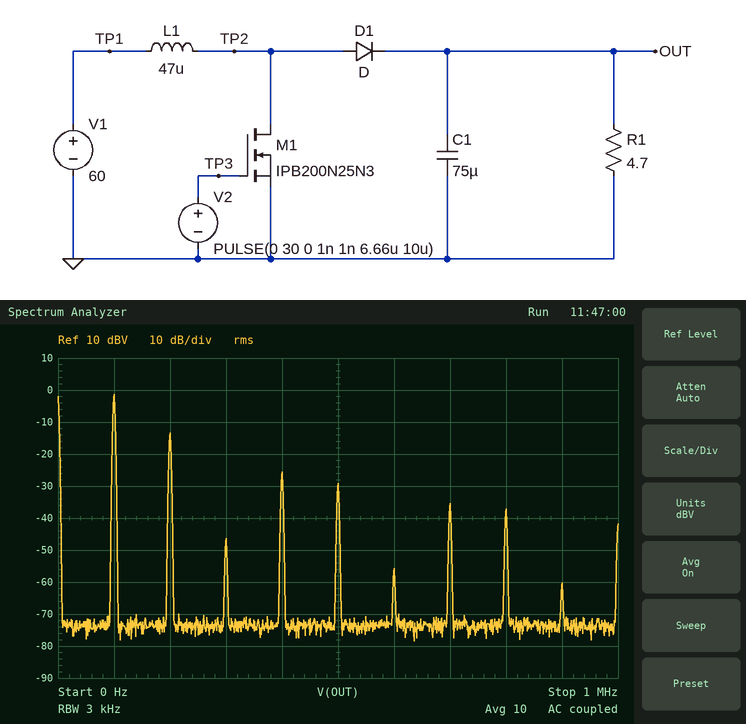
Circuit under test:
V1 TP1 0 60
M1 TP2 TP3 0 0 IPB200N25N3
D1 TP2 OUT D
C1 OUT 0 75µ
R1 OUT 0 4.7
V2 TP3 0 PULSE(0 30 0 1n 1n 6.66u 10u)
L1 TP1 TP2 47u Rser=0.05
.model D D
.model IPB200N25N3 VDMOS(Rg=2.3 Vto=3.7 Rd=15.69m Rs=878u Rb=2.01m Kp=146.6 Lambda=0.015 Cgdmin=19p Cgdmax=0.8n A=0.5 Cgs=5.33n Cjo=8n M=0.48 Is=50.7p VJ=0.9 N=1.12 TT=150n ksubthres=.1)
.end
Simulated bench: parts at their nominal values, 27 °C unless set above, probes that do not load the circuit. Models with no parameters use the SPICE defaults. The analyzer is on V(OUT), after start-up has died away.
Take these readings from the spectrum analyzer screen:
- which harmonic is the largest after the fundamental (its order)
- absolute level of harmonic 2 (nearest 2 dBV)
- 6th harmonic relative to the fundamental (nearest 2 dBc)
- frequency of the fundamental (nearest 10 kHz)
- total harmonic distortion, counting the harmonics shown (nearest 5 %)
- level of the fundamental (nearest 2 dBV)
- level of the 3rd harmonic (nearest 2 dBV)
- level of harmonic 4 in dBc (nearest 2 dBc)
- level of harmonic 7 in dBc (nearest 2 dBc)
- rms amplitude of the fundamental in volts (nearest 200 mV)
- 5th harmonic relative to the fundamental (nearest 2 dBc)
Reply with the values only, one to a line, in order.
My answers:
2
-14 dBV
-54 dBc
100 kHz
25 %
-2 dBV
-46 dBV
-24 dBc
-34 dBc
800 mV
-28 dBc
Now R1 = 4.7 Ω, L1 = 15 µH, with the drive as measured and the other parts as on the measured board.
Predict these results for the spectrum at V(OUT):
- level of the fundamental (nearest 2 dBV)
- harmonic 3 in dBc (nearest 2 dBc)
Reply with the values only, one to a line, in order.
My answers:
-2 dBV
-36 dBc
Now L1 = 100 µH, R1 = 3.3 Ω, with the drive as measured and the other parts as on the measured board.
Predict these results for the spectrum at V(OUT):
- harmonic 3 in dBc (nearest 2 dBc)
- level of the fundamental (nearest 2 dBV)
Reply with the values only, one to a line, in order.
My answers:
-50 dBc
2 dBV
